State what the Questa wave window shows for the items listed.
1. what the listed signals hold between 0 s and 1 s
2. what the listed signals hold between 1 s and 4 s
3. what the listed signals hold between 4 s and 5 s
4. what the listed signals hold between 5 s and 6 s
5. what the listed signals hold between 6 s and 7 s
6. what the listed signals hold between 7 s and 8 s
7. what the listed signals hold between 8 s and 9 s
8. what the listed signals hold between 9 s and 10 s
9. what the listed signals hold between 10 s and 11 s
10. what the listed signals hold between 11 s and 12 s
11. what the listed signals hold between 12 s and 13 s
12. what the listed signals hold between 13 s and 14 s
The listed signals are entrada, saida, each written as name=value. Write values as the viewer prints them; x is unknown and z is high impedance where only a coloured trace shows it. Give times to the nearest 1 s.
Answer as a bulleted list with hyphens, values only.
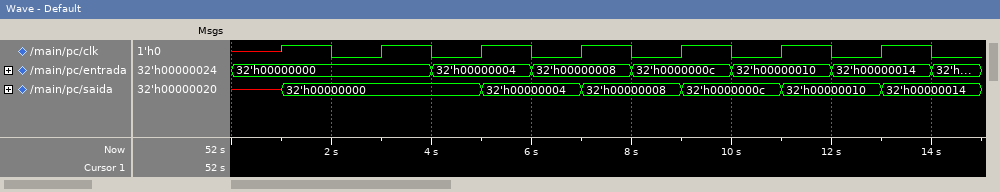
- entrada=32'h00000000, saida=x
- entrada=32'h00000000, saida=32'h00000000
- entrada=32'h00000004, saida=32'h00000000
- entrada=32'h00000004, saida=32'h00000004
- entrada=32'h00000008, saida=32'h00000004
- entrada=32'h00000008, saida=32'h00000008
- entrada=32'h0000000c, saida=32'h00000008
- entrada=32'h0000000c, saida=32'h0000000c
- entrada=32'h00000010, saida=32'h0000000c
- entrada=32'h00000010, saida=32'h00000010
- entrada=32'h00000014, saida=32'h00000010
- entrada=32'h00000014, saida=32'h00000014
